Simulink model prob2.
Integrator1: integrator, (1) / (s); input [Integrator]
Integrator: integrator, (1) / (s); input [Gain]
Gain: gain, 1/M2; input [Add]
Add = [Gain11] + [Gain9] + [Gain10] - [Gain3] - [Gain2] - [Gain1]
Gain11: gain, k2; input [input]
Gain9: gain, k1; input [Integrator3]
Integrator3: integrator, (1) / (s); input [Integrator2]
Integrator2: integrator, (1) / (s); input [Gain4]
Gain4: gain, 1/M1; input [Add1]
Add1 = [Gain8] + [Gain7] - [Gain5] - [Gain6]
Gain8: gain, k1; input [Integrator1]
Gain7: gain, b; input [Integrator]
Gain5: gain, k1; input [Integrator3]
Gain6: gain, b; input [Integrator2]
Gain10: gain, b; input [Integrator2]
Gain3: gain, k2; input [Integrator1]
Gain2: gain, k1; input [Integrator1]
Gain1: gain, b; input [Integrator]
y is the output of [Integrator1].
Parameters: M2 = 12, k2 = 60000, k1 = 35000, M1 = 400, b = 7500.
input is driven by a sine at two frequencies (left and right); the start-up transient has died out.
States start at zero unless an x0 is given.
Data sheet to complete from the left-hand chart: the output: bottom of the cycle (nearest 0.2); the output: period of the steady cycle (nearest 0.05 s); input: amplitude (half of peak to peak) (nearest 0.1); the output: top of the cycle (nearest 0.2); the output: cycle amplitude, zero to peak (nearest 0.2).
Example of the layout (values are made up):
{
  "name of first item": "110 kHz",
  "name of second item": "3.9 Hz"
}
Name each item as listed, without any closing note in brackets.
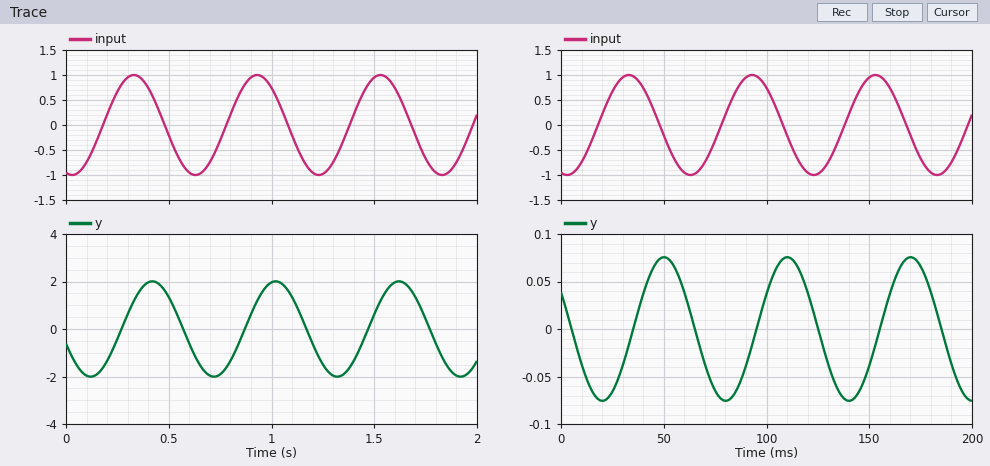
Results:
{
  "the output: bottom of the cycle": "-2.0",
  "the output: period of the steady cycle": "0.60 s",
  "input: amplitude (half of peak to peak)": "1.0",
  "the output: top of the cycle": "2.0",
  "the output: cycle amplitude, zero to peak": "2.0"
}
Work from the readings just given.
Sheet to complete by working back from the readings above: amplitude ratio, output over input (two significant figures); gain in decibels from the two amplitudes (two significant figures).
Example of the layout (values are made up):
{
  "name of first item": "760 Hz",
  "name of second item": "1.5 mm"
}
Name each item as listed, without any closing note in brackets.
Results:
{
  "amplitude ratio, output over input": "2.0",
  "gain in decibels from the two amplitudes": "6.0 dB"
}
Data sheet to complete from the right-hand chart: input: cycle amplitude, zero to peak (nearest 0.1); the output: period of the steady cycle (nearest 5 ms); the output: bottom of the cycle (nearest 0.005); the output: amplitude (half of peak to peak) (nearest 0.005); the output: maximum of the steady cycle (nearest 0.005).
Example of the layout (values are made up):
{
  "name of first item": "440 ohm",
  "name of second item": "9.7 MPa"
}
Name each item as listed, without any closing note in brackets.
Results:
{
  "input: cycle amplitude, zero to peak": "1.0",
  "the output: period of the steady cycle": "60 ms",
  "the output: bottom of the cycle": "-0.075",
  "the output: amplitude (half of peak to peak)": "0.075",
  "the output: maximum of the steady cycle": "0.075"
}
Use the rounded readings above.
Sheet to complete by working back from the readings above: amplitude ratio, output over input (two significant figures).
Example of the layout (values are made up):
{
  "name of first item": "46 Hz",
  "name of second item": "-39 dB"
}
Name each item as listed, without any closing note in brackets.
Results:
{
  "amplitude ratio, output over input": "0.075"
}
